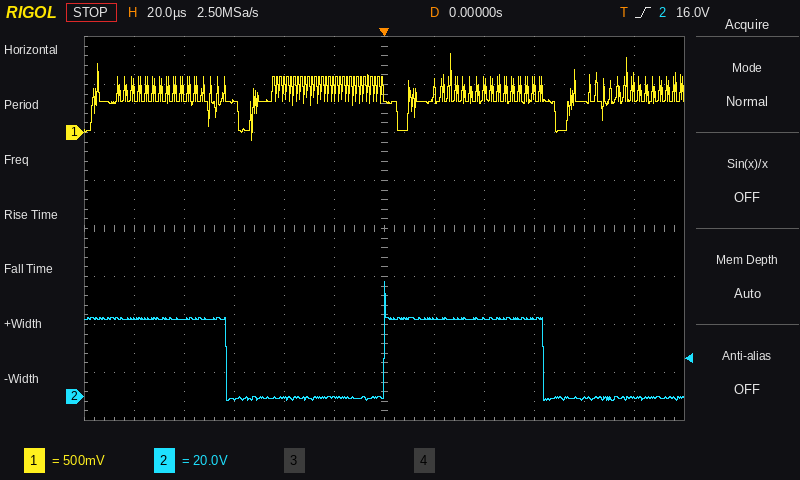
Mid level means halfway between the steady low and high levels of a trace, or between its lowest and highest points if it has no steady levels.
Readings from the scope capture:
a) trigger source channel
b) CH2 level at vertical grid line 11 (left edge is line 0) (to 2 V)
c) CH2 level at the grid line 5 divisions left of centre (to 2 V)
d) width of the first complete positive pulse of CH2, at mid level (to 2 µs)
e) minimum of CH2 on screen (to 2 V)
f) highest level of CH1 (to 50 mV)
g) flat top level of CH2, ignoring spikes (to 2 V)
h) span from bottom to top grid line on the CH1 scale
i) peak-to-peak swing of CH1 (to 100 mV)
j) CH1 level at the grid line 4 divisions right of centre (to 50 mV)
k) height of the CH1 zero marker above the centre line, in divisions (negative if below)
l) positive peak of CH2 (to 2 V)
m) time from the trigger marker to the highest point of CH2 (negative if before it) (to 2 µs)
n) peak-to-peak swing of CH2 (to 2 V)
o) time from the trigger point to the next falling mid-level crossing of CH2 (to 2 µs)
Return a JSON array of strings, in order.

["CH2", "0 V", "32 V", "64 µs", "-2 V", "800 mV", "32 V", "4 V", "900 mV", "300 mV", "+2.0 div", "48 V", "0 µs", "50 V", "64 µs"]
